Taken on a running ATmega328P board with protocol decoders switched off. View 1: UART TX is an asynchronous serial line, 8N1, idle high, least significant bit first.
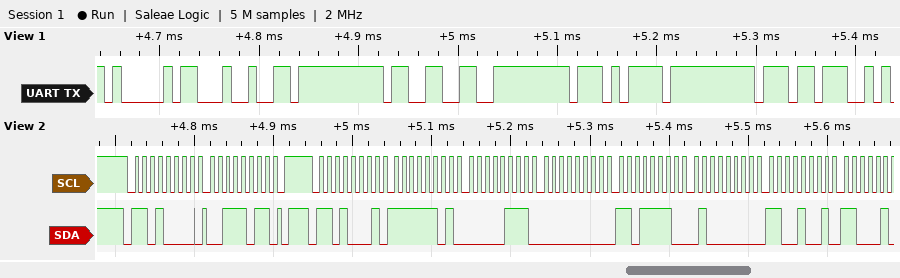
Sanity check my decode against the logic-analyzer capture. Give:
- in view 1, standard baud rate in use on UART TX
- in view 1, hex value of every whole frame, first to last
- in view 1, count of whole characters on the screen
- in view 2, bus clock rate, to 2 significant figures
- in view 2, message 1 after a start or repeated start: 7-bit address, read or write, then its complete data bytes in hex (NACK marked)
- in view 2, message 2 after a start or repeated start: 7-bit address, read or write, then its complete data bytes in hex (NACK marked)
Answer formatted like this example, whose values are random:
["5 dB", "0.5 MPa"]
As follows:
["115200 baud", "41 24 FF 33 FE D7 FF B7", "8", "100 kHz", "0x68 write: 3B", "0x68 read: FD 07 00 DE 40 C9"]
